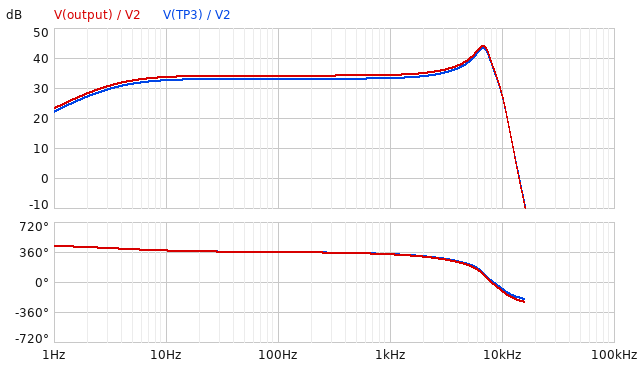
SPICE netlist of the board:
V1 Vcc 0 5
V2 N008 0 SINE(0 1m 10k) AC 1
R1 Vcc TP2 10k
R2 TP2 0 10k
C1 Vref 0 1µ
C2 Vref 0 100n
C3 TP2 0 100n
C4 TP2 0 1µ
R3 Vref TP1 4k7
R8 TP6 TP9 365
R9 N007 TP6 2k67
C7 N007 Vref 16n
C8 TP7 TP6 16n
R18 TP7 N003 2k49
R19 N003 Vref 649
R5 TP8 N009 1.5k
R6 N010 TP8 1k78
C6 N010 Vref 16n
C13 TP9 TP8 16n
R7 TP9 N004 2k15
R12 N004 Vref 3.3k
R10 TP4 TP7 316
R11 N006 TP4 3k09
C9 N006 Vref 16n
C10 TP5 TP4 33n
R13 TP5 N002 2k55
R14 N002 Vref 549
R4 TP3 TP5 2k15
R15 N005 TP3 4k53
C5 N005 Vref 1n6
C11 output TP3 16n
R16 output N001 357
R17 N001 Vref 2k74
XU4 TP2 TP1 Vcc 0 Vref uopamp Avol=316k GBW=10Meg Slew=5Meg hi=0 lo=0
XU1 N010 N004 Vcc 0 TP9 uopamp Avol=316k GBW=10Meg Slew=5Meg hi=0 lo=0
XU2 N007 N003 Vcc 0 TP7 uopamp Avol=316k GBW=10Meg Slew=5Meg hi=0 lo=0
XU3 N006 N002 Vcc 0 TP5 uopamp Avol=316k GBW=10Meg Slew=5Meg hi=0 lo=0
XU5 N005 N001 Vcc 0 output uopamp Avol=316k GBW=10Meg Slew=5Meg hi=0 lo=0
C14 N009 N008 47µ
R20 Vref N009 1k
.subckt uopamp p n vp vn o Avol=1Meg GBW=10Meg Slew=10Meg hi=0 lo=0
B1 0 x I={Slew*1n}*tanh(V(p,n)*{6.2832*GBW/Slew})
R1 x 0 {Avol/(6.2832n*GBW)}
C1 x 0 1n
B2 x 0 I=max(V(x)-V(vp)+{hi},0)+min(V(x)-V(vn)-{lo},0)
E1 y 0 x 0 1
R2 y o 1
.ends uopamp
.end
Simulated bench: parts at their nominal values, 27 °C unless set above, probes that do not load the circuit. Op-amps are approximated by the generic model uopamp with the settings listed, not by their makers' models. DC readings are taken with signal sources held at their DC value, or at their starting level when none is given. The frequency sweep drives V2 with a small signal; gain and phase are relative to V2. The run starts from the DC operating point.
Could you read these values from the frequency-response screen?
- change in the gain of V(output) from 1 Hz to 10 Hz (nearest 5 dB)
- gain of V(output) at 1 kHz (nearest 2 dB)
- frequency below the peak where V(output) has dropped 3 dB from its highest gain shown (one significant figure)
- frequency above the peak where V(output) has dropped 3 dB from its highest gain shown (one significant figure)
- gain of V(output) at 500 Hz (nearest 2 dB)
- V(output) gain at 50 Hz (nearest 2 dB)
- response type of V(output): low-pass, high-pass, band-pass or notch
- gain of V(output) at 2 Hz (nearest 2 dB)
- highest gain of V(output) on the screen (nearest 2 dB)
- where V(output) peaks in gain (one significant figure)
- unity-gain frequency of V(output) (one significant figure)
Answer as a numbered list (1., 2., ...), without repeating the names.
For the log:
1. 10 dB
2. 34 dB
3. 6 kHz
4. 8 kHz
5. 34 dB
6. 34 dB
7. band-pass
8. 28 dB
9. 44 dB
10. 7 kHz
11. 10 kHz
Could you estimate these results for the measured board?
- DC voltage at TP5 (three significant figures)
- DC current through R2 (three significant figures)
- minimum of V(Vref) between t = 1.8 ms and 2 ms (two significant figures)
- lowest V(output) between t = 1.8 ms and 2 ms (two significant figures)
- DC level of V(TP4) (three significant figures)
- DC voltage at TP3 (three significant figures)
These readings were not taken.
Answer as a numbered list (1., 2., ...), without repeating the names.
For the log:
1. 2.50 V
2. 250 µA
3. 2.5 V
4. 2.5 V
5. 2.50 V
6. 2.50 V
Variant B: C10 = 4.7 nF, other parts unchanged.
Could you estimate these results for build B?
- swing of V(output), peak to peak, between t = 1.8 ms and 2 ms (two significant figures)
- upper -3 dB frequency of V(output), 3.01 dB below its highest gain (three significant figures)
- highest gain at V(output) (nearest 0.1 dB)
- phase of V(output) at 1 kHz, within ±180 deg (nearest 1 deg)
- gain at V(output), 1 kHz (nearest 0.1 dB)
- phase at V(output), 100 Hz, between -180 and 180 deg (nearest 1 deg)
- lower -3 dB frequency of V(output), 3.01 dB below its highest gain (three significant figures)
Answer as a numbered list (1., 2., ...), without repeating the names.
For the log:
1. 18 mV
2. 3.58 kHz
3. 34.1 dB
4. -42 deg
5. 33.8 dB
6. -2 deg
7. 3.38 Hz
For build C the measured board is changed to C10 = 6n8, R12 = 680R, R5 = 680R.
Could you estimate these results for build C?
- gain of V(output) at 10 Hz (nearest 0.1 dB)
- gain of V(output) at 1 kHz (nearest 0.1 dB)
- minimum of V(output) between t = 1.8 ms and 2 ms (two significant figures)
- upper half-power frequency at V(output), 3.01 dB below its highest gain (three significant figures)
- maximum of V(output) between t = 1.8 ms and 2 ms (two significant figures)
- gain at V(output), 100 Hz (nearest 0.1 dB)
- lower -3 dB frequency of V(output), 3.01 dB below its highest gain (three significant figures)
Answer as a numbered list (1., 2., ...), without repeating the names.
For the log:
1. 41.7 dB
2. 42.0 dB
3. 2.3 V
4. 9.77 kHz
5. 2.7 V
6. 42.2 dB
7. 7.43 kHz
